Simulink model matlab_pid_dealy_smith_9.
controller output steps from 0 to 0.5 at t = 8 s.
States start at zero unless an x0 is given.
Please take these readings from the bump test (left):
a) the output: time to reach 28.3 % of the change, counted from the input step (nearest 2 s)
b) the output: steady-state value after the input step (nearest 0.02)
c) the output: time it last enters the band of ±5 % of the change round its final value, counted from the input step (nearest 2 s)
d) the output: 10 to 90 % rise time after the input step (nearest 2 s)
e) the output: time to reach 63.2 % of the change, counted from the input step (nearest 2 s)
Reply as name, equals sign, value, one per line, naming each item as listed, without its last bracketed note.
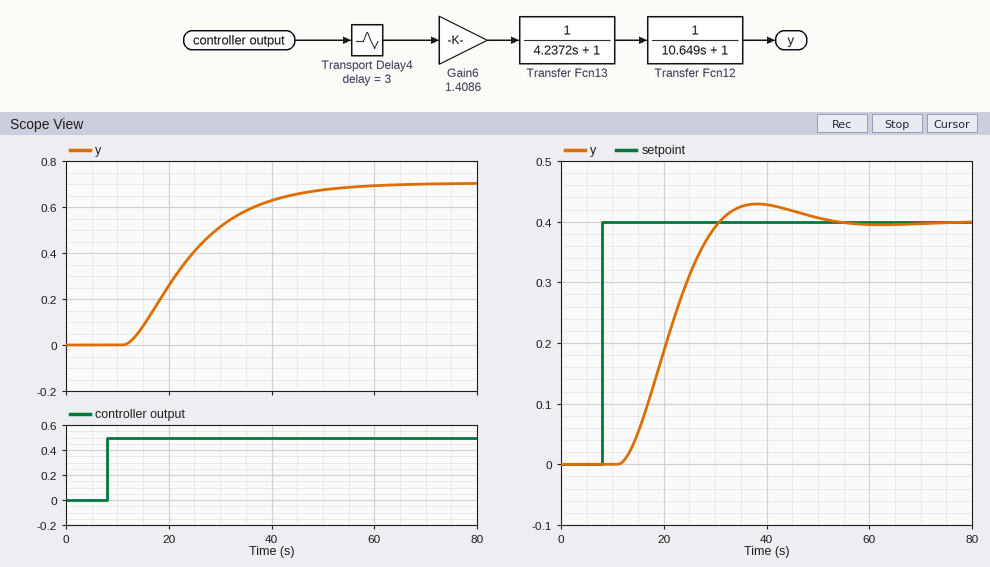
the output: time to reach 28.3 % of the change, counted from the input step = 10 s
the output: steady-state value after the input step = 0.70
the output: time it last enters the band of ±5 % of the change round its final value, counted from the input step = 40 s
the output: 10 to 90 % rise time after the input step = 26 s
the output: time to reach 63.2 % of the change, counted from the input step = 18 s
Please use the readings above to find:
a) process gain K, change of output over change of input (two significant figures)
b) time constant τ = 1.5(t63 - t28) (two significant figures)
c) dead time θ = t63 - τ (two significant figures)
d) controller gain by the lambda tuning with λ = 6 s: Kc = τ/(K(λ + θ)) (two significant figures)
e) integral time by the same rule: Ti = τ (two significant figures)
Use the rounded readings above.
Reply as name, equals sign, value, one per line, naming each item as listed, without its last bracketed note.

process gain K, change of output over change of input = 1.4
time constant τ = 1.5(t63 - t28) = 12 s
dead time θ = t63 - τ = 6.0 s
controller gain by the lambda tuning with λ = 6 s: Kc = τ/(K(λ + θ)) = 0.71
integral time by the same rule: Ti = τ = 12 s
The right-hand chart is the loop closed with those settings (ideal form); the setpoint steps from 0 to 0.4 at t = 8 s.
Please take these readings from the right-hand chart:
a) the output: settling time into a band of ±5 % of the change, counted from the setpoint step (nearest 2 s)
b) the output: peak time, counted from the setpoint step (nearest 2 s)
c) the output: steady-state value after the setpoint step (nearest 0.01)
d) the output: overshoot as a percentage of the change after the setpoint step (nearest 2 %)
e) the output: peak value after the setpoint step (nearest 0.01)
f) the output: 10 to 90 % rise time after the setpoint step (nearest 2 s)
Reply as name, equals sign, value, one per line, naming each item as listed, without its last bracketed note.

the output: settling time into a band of ±5 % of the change, counted from the setpoint step = 36 s
the output: peak time, counted from the setpoint step = 30 s
the output: steady-state value after the setpoint step = 0.40
the output: overshoot as a percentage of the change after the setpoint step = 8 %
the output: peak value after the setpoint step = 0.43
the output: 10 to 90 % rise time after the setpoint step = 14 s
